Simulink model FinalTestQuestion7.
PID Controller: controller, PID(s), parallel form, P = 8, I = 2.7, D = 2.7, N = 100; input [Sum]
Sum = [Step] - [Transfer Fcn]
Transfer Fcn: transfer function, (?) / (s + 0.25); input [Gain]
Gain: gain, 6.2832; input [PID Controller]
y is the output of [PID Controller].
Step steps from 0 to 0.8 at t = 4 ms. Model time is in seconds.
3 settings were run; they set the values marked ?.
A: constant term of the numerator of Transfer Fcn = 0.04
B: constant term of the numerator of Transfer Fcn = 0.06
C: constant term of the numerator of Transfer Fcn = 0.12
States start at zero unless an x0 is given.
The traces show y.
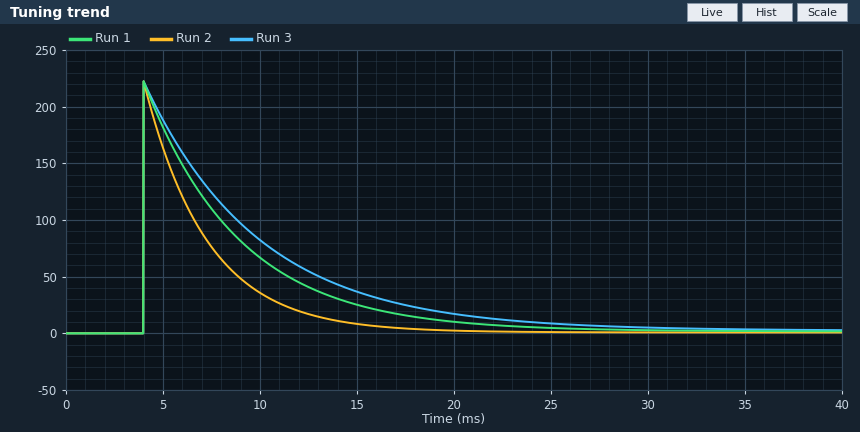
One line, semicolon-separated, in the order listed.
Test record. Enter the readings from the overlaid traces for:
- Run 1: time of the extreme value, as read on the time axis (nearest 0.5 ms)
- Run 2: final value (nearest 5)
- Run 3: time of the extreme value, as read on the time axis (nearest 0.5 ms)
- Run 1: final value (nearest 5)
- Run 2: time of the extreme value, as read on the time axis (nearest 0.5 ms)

4.0 ms; 0; 4.0 ms; 0; 4.0 ms
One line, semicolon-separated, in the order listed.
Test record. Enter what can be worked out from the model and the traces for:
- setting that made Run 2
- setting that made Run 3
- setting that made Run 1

C; A; B
